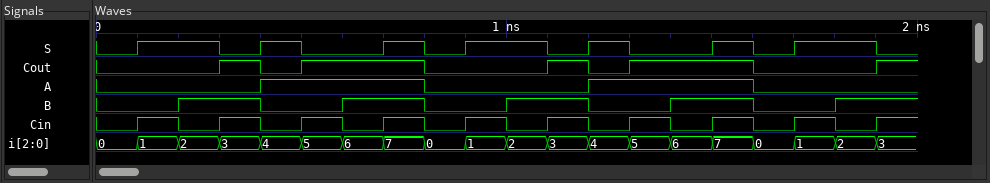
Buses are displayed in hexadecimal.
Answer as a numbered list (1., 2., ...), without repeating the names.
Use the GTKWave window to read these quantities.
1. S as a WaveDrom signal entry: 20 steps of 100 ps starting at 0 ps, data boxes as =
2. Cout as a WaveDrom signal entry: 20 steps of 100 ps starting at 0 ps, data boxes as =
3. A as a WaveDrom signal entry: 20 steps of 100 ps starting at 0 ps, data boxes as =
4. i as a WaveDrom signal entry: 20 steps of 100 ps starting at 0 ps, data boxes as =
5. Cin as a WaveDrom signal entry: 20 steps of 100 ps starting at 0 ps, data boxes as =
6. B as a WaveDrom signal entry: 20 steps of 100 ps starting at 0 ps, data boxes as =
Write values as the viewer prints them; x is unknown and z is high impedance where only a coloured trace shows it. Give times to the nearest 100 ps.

1. {name: 'S', wave: '01.010.101.010.101.0'}
2. {name: 'Cout', wave: '0..101..0..101..0..1'}
3. {name: 'A', wave: '0...1...0...1...0...'}
4. {name: 'i', wave: '====================', data: '0 1 2 3 4 5 6 7 0 1 2 3 4 5 6 7 0 1 2 3'}
5. {name: 'Cin', wave: '01010101010101010101'}
6. {name: 'B', wave: '0.1.0.1.0.1.0.1.0.1.'}
